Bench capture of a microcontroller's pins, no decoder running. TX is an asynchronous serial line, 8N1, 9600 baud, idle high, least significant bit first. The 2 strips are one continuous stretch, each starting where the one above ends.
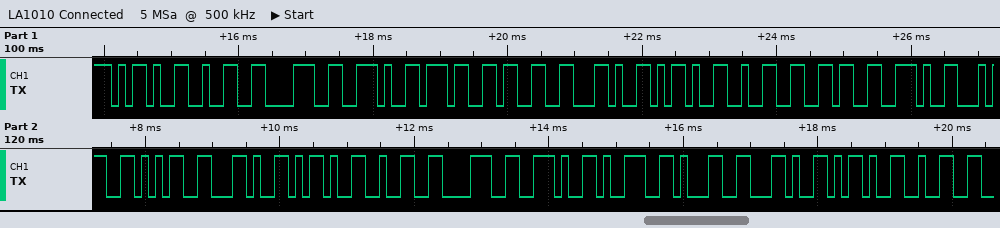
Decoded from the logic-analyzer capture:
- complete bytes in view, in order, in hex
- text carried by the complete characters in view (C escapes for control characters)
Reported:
2D 32 38 2E 37 33 2C 2D 32 36 2E 34 35 2C 2D 32 38 2E 39 31 2C 2D 32
"-28.73,-26.45,-28.91,-2"
